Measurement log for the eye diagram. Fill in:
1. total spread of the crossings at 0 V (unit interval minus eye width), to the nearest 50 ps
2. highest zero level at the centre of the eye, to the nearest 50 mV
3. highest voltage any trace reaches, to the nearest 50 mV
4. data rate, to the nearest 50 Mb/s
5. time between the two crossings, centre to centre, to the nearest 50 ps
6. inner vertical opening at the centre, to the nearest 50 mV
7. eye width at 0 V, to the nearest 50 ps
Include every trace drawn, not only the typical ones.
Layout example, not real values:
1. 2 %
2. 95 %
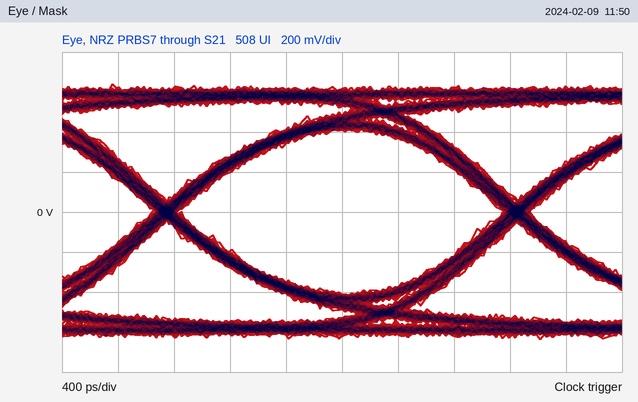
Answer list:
1. 200 ps
2. -400 mV
3. 650 mV
4. 400 Mb/s
5. 2.50 ns
6. 800 mV
7. 2.30 ns
